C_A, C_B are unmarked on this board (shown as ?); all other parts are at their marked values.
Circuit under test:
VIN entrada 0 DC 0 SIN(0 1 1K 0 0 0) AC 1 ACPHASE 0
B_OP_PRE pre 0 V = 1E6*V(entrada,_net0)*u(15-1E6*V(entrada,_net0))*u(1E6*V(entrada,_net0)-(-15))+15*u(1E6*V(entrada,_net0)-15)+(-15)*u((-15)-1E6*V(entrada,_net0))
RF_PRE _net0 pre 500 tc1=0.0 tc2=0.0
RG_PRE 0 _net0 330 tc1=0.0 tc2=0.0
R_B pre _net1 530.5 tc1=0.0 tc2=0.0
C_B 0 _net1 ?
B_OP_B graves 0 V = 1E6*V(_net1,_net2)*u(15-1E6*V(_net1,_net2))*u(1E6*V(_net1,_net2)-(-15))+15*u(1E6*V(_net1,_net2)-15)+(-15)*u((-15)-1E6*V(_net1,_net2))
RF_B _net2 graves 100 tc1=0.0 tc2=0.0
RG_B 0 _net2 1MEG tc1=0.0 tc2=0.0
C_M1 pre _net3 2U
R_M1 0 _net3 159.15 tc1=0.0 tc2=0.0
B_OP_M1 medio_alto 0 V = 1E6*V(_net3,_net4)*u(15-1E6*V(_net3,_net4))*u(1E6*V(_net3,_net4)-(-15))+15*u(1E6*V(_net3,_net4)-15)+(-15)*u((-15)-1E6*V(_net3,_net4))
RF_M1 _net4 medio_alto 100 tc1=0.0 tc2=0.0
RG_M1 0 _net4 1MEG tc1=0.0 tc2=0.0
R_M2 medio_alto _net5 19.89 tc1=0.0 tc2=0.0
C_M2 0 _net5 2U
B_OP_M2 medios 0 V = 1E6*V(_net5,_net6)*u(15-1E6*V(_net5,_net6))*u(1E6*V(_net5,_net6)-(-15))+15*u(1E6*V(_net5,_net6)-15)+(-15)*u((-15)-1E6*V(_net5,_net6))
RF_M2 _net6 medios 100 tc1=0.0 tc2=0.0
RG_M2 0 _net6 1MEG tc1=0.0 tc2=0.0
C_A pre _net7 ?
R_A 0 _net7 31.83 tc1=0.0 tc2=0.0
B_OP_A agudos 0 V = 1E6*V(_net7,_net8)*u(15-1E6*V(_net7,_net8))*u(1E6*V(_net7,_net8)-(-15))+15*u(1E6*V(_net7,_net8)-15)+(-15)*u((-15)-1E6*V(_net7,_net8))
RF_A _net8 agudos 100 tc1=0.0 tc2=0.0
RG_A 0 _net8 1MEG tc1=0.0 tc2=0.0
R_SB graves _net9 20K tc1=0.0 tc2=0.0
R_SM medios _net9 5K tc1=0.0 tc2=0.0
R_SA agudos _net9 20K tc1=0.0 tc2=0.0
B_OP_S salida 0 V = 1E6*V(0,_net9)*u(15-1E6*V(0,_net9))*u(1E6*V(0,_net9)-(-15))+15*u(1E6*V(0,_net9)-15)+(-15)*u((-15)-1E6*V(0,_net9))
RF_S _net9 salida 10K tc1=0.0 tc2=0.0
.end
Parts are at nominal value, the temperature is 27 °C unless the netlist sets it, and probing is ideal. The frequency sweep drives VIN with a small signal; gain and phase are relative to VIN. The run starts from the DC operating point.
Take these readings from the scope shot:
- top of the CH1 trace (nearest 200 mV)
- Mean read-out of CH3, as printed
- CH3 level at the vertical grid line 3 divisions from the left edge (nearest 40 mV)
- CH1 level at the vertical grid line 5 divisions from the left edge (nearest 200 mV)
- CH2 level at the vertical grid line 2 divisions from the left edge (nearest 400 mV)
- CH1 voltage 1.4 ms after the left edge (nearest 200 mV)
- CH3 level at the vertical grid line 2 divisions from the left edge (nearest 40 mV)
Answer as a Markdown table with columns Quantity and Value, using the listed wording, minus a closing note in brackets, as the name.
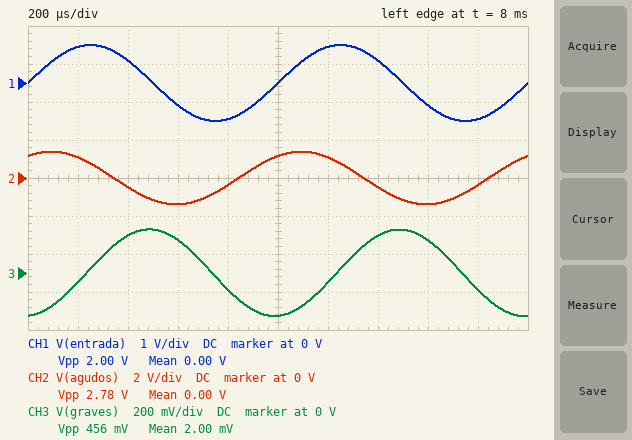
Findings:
| Quantity | Value |
|---|---|
| top of the CH1 trace | 1.0 V |
| Mean read-out of CH3, as printed | 2.00 mV |
| CH3 level at the vertical grid line 3 divisions from the left edge | 160 mV |
| CH1 level at the vertical grid line 5 divisions from the left edge | 0 V |
| CH2 level at the vertical grid line 2 divisions from the left edge | -400 mV |
| CH1 voltage 1.4 ms after the left edge | 600 mV |
| CH3 level at the vertical grid line 2 divisions from the left edge | 200 mV |
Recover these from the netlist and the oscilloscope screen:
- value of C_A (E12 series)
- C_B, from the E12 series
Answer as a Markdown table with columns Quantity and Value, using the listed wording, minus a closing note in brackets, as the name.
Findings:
| Quantity | Value |
|---|---|
| value of C_A | 3.3 µF |
| C_B, from the E12 series | 3.3 µF |
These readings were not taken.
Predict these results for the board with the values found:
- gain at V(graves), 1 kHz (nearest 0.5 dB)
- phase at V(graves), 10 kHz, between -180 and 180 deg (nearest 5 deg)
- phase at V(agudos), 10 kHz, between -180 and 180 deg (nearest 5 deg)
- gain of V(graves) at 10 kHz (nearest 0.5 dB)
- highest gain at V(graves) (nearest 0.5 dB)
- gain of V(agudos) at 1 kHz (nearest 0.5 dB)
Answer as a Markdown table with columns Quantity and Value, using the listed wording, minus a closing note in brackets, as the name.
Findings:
| Quantity | Value |
|---|---|
| gain at V(graves), 1 kHz | -13.0 dB |
| phase at V(graves), 10 kHz, between -180 and 180 deg | -90 deg |
| phase at V(agudos), 10 kHz, between -180 and 180 deg | 10 deg |
| gain of V(graves) at 10 kHz | -33.0 dB |
| highest gain at V(graves) | 8.0 dB |
| gain of V(agudos) at 1 kHz | 3.0 dB |
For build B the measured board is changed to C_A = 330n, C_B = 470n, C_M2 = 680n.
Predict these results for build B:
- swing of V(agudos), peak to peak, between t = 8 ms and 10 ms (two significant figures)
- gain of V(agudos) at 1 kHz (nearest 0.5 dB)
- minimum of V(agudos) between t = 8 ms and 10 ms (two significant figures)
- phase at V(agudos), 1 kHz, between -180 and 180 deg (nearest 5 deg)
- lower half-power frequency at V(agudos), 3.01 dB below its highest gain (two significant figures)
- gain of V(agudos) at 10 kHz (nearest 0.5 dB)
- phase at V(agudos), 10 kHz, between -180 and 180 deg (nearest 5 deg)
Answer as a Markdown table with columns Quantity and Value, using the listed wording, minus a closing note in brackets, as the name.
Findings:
| Quantity | Value |
|---|---|
| swing of V(agudos), peak to peak, between t = 8 ms and 10 ms | 330 mV |
| gain of V(agudos) at 1 kHz | -15.5 dB |
| minimum of V(agudos) between t = 8 ms and 10 ms | -170 mV |
| phase at V(agudos), 1 kHz, between -180 and 180 deg | 85 deg |
| lower half-power frequency at V(agudos), 3.01 dB below its highest gain | 15 kHz |
| gain of V(agudos) at 10 kHz | 3.0 dB |
| phase at V(agudos), 10 kHz, between -180 and 180 deg | 55 deg |
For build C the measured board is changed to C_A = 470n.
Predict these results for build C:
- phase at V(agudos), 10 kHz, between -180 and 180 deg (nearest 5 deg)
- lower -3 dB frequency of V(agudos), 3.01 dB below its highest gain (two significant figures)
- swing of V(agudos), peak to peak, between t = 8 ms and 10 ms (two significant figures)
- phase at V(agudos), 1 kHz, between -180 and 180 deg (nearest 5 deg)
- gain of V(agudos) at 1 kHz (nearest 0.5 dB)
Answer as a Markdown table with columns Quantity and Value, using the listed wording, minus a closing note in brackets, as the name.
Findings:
| Quantity | Value |
|---|---|
| phase at V(agudos), 10 kHz, between -180 and 180 deg | 45 deg |
| lower -3 dB frequency of V(agudos), 3.01 dB below its highest gain | 11 kHz |
| swing of V(agudos), peak to peak, between t = 8 ms and 10 ms | 470 mV |
| phase at V(agudos), 1 kHz, between -180 and 180 deg | 85 deg |
| gain of V(agudos) at 1 kHz | -12.5 dB |
